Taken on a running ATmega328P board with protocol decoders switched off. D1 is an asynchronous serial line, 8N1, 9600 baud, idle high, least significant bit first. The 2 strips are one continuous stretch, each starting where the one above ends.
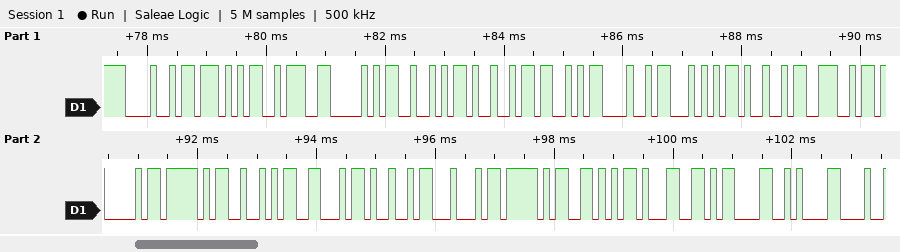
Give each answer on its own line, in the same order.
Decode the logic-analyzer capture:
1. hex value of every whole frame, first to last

48 57 3A 50 52 49 53 48 54 49 4E 41 5F 52 46 49 44 5F 56 31 0D 0A
